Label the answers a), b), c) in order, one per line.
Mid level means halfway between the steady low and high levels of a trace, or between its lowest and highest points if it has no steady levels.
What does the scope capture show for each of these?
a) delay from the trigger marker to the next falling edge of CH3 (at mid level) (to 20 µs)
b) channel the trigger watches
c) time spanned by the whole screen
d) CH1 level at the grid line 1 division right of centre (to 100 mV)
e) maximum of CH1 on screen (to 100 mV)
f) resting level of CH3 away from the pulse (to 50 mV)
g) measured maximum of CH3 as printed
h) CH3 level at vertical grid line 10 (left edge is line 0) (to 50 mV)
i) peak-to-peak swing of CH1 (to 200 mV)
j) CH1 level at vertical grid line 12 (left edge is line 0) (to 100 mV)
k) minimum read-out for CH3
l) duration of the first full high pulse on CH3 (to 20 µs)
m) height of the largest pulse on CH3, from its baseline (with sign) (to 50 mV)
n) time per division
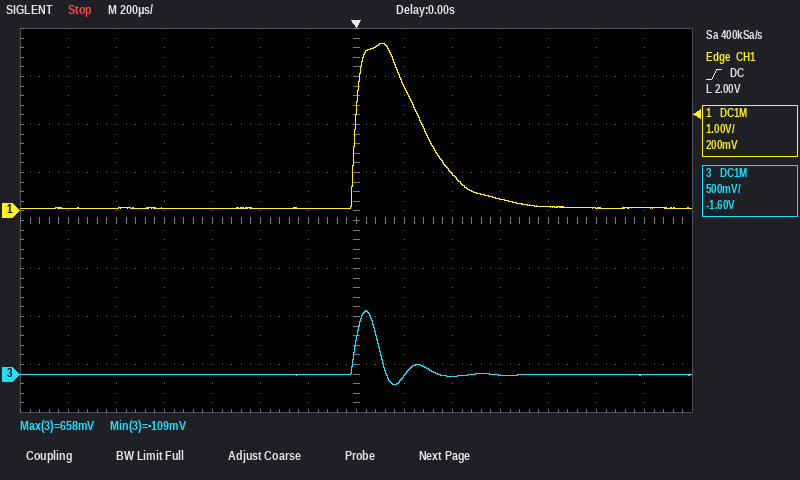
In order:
a) 100 µs
b) CH1
c) 2.8 ms
d) 2.6 V
e) 3.5 V
f) 0 mV
g) 658 mV
h) 0 mV
i) 3.4 V
j) 100 mV
k) -109 mV
l) 100 µs
m) +650 mV
n) 200 µs
